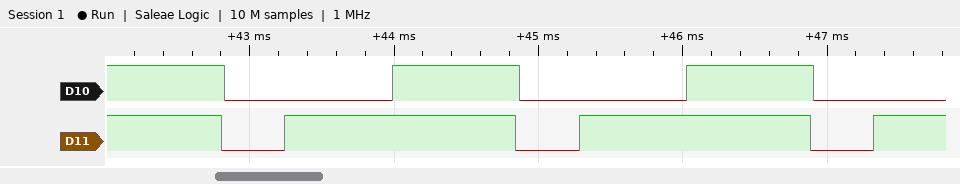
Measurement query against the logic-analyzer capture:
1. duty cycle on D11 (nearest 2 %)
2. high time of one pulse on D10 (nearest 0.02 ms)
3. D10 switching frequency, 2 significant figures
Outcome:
78 %
0.88 ms
490 Hz
